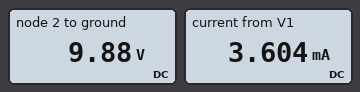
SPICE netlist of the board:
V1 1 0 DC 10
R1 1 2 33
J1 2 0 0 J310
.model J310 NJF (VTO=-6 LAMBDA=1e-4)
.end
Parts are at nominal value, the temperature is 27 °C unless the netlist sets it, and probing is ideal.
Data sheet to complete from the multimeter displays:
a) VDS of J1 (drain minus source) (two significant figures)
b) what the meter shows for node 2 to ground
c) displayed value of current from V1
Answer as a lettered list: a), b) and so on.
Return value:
a) 9.9 V
b) 9.88 V
c) 3.604 mA
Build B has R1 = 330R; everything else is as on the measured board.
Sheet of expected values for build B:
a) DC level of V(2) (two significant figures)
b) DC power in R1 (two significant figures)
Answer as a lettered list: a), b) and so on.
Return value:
a) 8.8 V
b) 4.3 mW
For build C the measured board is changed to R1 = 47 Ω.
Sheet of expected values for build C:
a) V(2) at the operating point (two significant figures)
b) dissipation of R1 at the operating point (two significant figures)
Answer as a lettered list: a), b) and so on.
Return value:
a) 9.8 V
b) 610 µW
